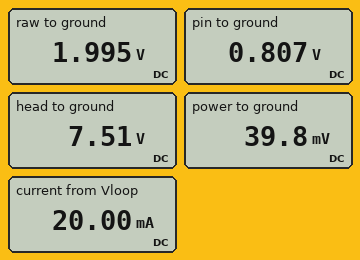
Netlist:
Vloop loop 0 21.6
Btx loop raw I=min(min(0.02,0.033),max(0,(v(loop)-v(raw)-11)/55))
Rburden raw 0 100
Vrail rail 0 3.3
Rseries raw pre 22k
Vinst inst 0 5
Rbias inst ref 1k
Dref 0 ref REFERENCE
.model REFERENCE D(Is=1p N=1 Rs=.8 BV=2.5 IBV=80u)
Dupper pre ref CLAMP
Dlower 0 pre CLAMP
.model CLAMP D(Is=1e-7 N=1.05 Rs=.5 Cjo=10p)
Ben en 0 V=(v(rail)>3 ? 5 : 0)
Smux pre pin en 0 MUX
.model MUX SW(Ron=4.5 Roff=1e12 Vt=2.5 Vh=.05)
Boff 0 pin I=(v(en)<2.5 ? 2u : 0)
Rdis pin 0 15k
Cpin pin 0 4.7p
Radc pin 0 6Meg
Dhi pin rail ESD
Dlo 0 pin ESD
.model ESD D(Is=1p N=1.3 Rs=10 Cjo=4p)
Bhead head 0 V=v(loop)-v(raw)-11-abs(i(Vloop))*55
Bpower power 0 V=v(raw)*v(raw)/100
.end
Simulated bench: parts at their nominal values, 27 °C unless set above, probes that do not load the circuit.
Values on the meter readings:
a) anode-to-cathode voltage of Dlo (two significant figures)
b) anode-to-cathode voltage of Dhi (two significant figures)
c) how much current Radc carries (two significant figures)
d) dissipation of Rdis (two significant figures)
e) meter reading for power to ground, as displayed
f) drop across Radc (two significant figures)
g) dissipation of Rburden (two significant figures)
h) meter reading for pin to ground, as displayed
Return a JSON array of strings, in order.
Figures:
["-810 mV", "-2.5 V", "130 nA", "43 µW", "39.8 mV", "810 mV", "40 mW", "0.807 V"]
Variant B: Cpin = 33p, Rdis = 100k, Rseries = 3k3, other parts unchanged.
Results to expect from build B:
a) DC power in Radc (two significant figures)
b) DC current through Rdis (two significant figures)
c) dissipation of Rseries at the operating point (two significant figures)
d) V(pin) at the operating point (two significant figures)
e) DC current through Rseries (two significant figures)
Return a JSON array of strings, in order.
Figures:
["620 nW", "19 µA", "1.3 µW", "1.9 V", "20 µA"]
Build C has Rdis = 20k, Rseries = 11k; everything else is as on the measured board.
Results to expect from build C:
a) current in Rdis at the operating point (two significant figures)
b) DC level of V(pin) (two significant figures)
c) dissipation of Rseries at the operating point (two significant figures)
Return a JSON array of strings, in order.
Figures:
["64 µA", "1.3 V", "46 µW"]
